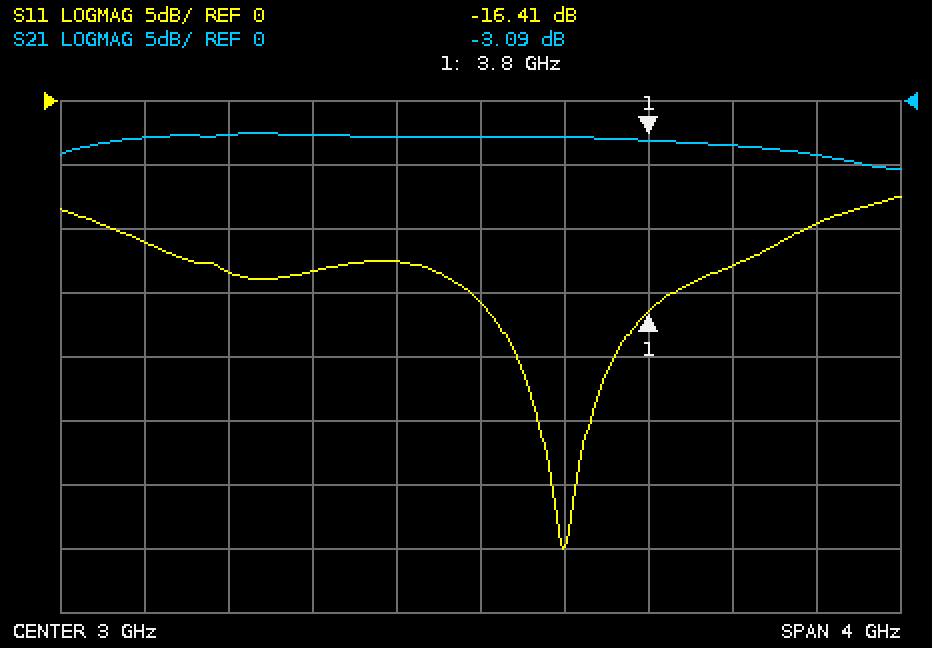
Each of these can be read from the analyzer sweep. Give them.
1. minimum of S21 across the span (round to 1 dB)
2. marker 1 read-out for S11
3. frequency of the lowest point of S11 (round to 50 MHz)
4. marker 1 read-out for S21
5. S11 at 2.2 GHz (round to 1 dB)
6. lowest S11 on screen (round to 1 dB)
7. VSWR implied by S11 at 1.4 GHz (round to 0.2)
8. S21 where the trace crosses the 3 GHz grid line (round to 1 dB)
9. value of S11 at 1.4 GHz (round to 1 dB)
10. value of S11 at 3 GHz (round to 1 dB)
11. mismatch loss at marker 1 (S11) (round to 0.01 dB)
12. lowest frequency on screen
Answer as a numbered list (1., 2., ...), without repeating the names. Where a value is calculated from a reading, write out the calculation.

1. -5 dB
2. -16.41 dB
3. 3.40 GHz
4. -3.09 dB
5. -13 dB
6. -35 dB
7. |Γ| = 10^(-11/20) = 0.2818; VSWR = (1 + 0.2818)/(1 − 0.2818) ≈ 1.8
8. -3 dB
9. -11 dB
10. -16 dB
11. −10 log10(1 − 10^(-16.41/10)) ≈ 0.10 dB
12. 1 GHz
